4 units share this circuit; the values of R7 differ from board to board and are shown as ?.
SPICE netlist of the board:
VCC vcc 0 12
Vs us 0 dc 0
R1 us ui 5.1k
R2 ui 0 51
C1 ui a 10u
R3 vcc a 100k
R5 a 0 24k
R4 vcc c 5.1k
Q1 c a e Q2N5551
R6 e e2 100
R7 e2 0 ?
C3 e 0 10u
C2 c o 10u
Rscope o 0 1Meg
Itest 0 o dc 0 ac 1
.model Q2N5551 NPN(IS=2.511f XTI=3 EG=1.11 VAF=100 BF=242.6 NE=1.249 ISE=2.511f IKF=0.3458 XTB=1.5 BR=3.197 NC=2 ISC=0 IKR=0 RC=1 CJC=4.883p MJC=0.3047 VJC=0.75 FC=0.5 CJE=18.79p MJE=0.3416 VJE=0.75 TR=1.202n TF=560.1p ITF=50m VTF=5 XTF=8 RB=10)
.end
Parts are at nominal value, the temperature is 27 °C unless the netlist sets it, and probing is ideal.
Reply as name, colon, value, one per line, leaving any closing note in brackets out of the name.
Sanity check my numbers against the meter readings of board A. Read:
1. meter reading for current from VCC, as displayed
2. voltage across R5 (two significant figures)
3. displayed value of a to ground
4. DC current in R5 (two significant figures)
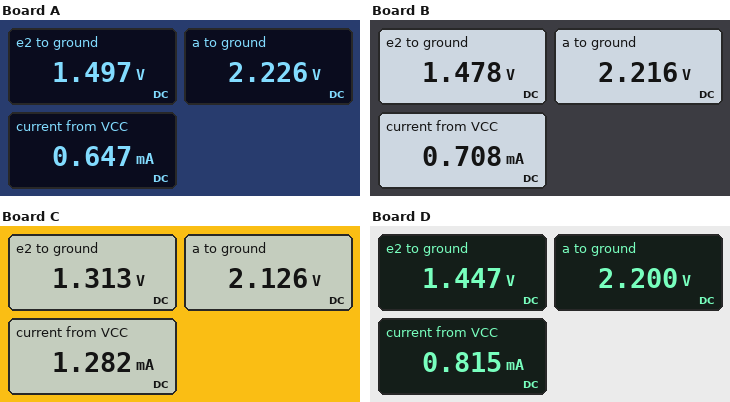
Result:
meter reading for current from VCC, as displayed: 0.647 mA
voltage across R5: 2.2 V
displayed value of a to ground: 2.226 V
DC current in R5: 93 µA
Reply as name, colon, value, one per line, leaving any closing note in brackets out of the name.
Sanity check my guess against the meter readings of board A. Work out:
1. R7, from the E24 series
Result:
R7, from the E24 series: 2.7 kΩ
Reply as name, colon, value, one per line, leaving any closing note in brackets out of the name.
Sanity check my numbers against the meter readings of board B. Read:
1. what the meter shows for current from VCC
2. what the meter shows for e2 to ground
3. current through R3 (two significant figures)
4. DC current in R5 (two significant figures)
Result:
what the meter shows for current from VCC: 0.708 mA
what the meter shows for e2 to ground: 1.478 V
current through R3: 98 µA
DC current in R5: 92 µA
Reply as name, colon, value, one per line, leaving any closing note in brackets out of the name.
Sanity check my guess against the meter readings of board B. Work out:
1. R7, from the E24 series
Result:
R7, from the E24 series: 2.4 kΩ
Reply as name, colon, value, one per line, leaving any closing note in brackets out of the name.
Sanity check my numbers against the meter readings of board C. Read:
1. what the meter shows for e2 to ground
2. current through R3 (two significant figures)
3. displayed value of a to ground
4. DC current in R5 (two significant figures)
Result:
what the meter shows for e2 to ground: 1.313 V
current through R3: 99 µA
displayed value of a to ground: 2.126 V
DC current in R5: 89 µA
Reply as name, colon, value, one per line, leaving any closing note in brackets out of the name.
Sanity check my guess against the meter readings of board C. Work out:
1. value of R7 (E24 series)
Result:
value of R7: 1.1 kΩ
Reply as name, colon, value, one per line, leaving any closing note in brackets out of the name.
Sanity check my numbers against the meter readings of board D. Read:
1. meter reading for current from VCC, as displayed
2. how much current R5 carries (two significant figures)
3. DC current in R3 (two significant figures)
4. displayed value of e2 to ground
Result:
meter reading for current from VCC, as displayed: 0.815 mA
how much current R5 carries: 92 µA
DC current in R3: 98 µA
displayed value of e2 to ground: 1.447 V
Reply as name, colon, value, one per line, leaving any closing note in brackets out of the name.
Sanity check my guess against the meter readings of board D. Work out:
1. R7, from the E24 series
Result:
R7, from the E24 series: 2 kΩ
